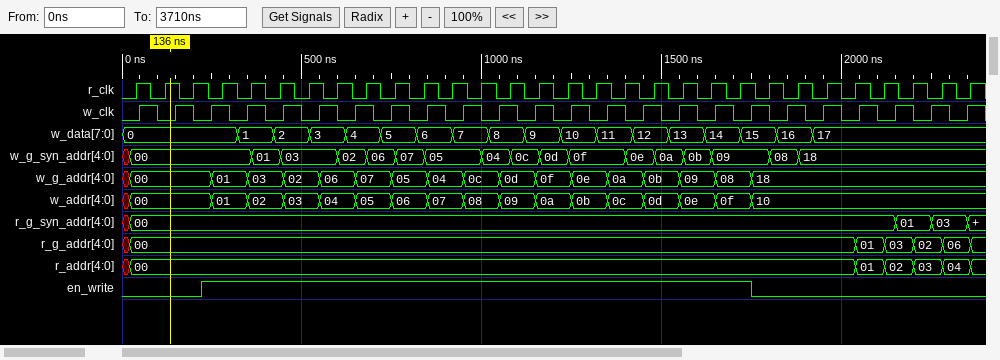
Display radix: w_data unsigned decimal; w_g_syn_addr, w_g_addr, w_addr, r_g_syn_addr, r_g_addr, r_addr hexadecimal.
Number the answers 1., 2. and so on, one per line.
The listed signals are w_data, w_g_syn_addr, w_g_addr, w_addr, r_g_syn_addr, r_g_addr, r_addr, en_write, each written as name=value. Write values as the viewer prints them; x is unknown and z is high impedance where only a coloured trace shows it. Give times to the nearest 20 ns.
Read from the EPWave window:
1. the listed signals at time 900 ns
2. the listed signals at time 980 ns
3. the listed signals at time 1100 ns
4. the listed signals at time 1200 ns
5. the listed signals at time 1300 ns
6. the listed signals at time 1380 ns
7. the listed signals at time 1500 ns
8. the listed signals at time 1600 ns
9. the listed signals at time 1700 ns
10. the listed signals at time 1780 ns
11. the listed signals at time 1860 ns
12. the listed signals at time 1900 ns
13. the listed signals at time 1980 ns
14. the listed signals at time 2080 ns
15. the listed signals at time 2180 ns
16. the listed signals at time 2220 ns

1. w_data=6, w_g_syn_addr=05, w_g_addr=04, w_addr=07, r_g_syn_addr=00, r_g_addr=00, r_addr=00, en_write=1
2. w_data=7, w_g_syn_addr=05, w_g_addr=0c, w_addr=08, r_g_syn_addr=00, r_g_addr=00, r_addr=00, en_write=1
3. w_data=8, w_g_syn_addr=0c, w_g_addr=0d, w_addr=09, r_g_syn_addr=00, r_g_addr=00, r_addr=00, en_write=1
4. w_data=9, w_g_syn_addr=0d, w_g_addr=0f, w_addr=0a, r_g_syn_addr=00, r_g_addr=00, r_addr=00, en_write=1
5. w_data=10, w_g_syn_addr=0f, w_g_addr=0e, w_addr=0b, r_g_syn_addr=00, r_g_addr=00, r_addr=00, en_write=1
6. w_data=11, w_g_syn_addr=0f, w_g_addr=0a, w_addr=0c, r_g_syn_addr=00, r_g_addr=00, r_addr=00, en_write=1
7. w_data=12, w_g_syn_addr=0a, w_g_addr=0b, w_addr=0d, r_g_syn_addr=00, r_g_addr=00, r_addr=00, en_write=1
8. w_data=13, w_g_syn_addr=0b, w_g_addr=09, w_addr=0e, r_g_syn_addr=00, r_g_addr=00, r_addr=00, en_write=1
9. w_data=14, w_g_syn_addr=09, w_g_addr=08, w_addr=0f, r_g_syn_addr=00, r_g_addr=00, r_addr=00, en_write=1
10. w_data=15, w_g_syn_addr=09, w_g_addr=18, w_addr=10, r_g_syn_addr=00, r_g_addr=00, r_addr=00, en_write=0
11. w_data=16, w_g_syn_addr=08, w_g_addr=18, w_addr=10, r_g_syn_addr=00, r_g_addr=00, r_addr=00, en_write=0
12. w_data=16, w_g_syn_addr=18, w_g_addr=18, w_addr=10, r_g_syn_addr=00, r_g_addr=00, r_addr=00, en_write=0
13. w_data=17, w_g_syn_addr=18, w_g_addr=18, w_addr=10, r_g_syn_addr=00, r_g_addr=00, r_addr=00, en_write=0
14. w_data=17, w_g_syn_addr=18, w_g_addr=18, w_addr=10, r_g_syn_addr=00, r_g_addr=01, r_addr=01, en_write=0
15. w_data=17, w_g_syn_addr=18, w_g_addr=18, w_addr=10, r_g_syn_addr=01, r_g_addr=03, r_addr=02, en_write=0
16. w_data=17, w_g_syn_addr=18, w_g_addr=18, w_addr=10, r_g_syn_addr=01, r_g_addr=02, r_addr=03, en_write=0
